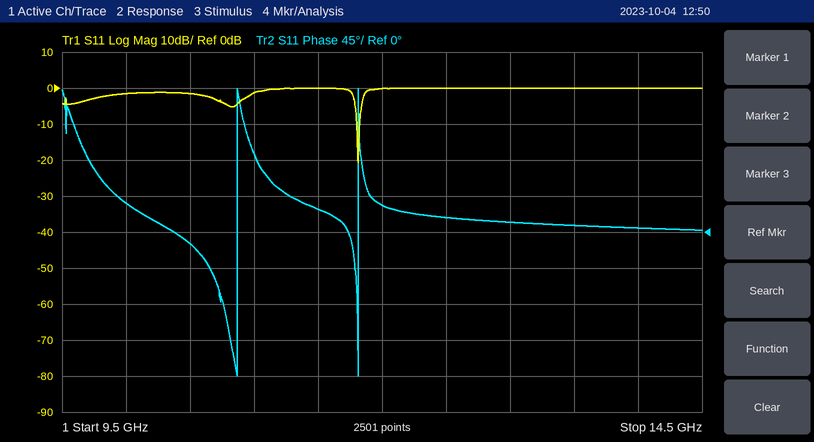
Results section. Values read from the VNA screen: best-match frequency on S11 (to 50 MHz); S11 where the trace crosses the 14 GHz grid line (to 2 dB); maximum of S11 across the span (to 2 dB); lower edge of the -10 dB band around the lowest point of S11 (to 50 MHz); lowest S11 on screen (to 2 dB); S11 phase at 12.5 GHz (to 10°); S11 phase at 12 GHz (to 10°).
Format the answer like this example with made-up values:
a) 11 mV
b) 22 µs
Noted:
a) 11.80 GHz
b) 0 dB
c) 0 dB
d) 11.80 GHz
e) -20 dB
f) 20°
g) 30°
